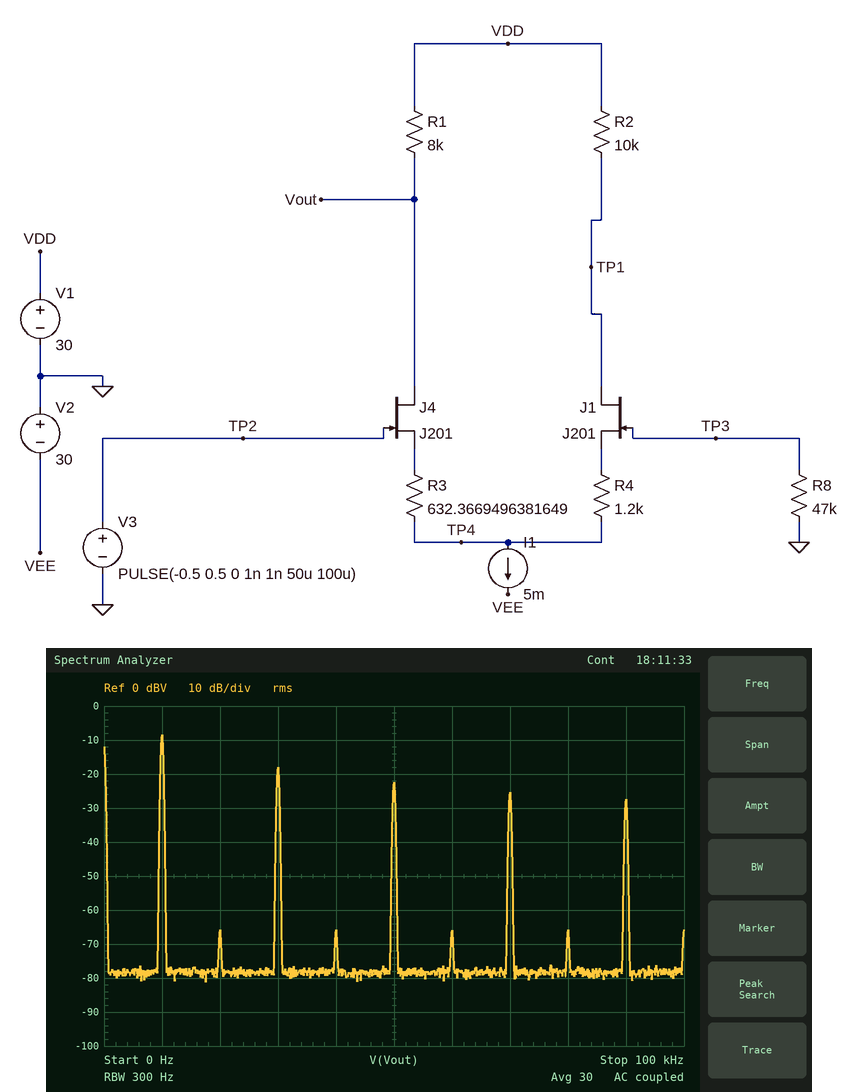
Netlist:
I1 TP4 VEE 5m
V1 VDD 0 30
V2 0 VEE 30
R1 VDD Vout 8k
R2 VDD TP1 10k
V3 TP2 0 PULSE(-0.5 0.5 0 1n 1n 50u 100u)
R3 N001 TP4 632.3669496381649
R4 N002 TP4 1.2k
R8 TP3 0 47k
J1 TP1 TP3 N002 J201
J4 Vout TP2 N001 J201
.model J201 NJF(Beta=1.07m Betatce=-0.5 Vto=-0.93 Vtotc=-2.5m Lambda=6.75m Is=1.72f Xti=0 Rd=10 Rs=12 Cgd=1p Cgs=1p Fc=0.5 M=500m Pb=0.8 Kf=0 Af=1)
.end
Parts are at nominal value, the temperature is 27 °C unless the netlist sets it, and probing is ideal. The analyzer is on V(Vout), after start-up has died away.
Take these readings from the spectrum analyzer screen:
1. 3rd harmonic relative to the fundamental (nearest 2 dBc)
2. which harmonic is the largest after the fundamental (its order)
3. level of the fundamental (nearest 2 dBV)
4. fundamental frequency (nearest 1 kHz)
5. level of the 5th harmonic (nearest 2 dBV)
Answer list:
-10 dBc
3
-8 dBV
10 kHz
-22 dBV
